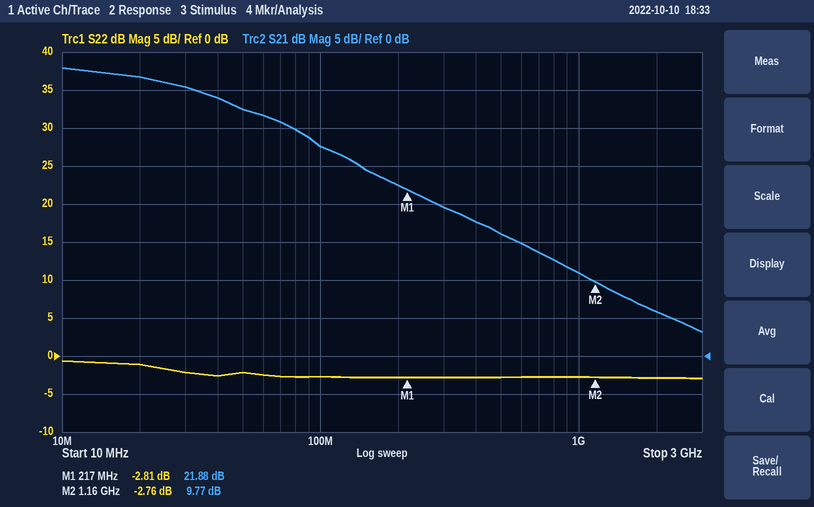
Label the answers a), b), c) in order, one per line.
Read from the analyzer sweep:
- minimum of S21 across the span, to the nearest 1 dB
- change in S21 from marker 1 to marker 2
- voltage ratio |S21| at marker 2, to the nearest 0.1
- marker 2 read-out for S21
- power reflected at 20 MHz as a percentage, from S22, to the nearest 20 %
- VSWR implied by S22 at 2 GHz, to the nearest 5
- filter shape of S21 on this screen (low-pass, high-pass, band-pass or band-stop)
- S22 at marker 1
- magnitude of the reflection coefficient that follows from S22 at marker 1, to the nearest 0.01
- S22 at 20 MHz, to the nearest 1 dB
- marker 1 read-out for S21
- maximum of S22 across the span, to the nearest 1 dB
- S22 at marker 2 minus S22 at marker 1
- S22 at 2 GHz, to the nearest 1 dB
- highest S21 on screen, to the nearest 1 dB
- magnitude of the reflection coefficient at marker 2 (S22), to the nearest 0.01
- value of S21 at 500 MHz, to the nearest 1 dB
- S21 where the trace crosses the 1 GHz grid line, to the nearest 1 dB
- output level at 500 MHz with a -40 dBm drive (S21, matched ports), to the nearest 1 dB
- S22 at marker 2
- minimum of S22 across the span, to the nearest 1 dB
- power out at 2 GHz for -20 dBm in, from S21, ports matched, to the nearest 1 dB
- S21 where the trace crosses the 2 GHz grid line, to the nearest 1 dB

a) 3 dB
b) -12.11 dB
c) 3.1
d) 9.77 dB
e) 80 %
f) 5
g) low-pass
h) -2.81 dB
i) 0.72
j) -1 dB
k) 21.88 dB
l) -1 dB
m) 0.05 dB
n) -3 dB
o) 38 dB
p) 0.73
q) 16 dB
r) 11 dB
s) -24 dBm
t) -2.76 dB
u) -3 dB
v) -14 dBm
w) 6 dB
